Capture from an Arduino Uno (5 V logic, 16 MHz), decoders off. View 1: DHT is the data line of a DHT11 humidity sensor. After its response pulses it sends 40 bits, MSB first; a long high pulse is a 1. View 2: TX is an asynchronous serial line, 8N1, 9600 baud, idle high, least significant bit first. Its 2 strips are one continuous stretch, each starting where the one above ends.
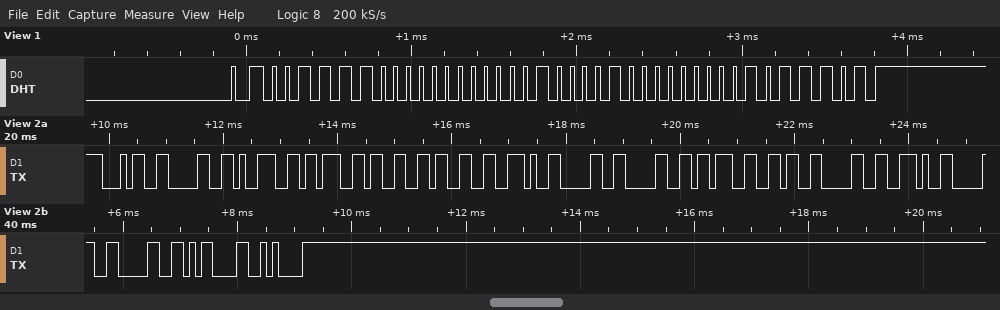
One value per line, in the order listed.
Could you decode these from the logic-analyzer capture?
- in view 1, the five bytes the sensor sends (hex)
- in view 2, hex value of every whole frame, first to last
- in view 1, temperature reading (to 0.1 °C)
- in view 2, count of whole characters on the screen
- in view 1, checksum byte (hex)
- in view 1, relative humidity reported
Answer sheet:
3C 00 21 00 5D
34 30 39 3B 33 33 2E 30 30 3B 36 30 2E 30 30 0D 0A
33.0 °C
17
0x5D
60 %
